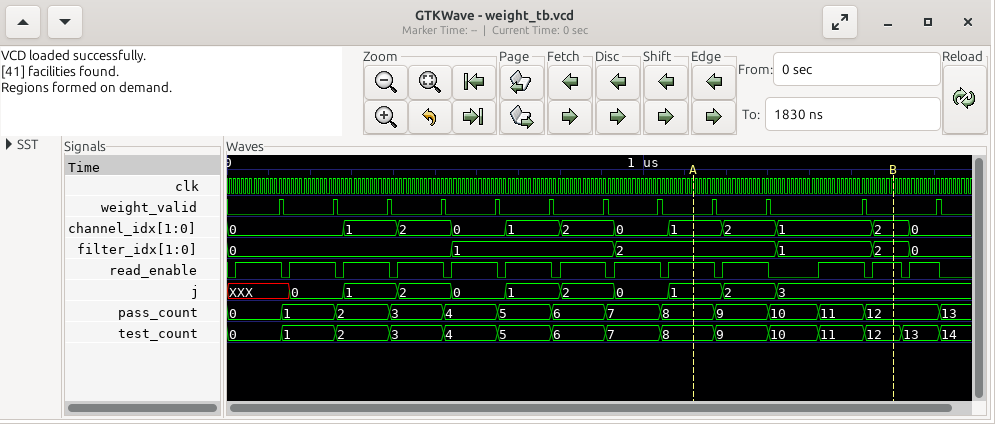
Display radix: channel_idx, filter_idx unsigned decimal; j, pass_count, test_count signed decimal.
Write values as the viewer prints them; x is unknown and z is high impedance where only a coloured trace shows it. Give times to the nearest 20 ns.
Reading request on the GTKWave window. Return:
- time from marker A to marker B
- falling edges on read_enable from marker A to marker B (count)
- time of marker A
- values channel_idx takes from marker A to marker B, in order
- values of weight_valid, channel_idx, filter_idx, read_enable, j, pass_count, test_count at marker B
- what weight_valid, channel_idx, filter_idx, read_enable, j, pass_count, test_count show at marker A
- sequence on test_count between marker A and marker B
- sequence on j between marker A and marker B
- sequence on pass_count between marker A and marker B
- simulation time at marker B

480 ns
3
1120 ns
1, 2, 1, 2
weight_valid=0, channel_idx=2, filter_idx=2, read_enable=1, j=3, pass_count=12, test_count=12
weight_valid=0, channel_idx=1, filter_idx=2, read_enable=1, j=1, pass_count=8, test_count=8
8, 9, 10, 11, 12
1, 2, 3
8, 9, 10, 11, 12
1600 ns
